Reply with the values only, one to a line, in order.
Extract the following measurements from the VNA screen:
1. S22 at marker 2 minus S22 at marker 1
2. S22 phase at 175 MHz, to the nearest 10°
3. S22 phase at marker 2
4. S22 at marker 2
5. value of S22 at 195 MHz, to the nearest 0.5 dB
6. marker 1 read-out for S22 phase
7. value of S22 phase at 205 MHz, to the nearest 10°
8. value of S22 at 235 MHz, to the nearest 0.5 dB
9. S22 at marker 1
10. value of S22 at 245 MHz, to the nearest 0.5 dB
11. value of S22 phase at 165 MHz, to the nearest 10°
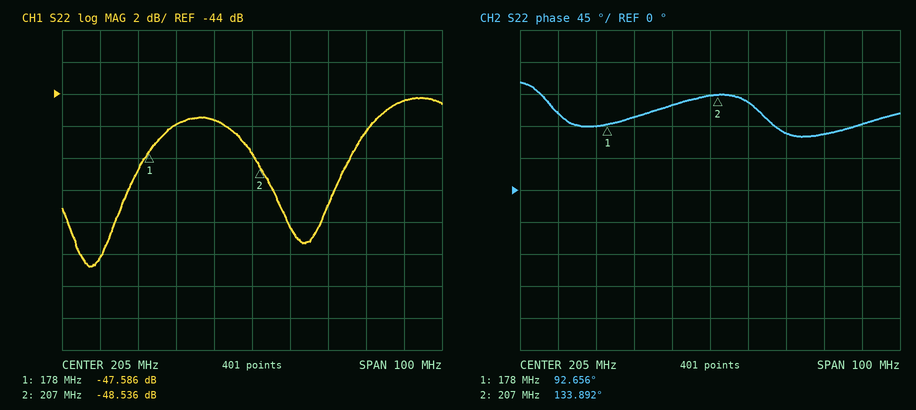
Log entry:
-0.950 dB
90°
133.892°
-48.536 dB
-45.5 dB
92.656°
130°
-46.5 dB
-47.586 dB
-44.5 dB
110°
